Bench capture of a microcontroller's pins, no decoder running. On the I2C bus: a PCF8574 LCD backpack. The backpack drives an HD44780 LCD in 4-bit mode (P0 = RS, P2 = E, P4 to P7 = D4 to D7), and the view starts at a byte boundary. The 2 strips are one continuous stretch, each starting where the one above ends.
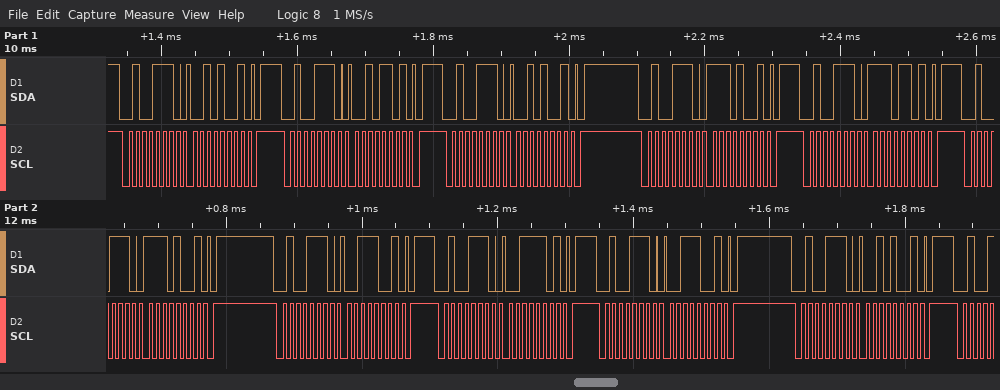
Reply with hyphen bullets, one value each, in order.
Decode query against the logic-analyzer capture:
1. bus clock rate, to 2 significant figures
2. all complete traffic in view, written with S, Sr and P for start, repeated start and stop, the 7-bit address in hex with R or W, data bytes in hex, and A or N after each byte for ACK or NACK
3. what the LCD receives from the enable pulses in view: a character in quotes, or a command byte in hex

- 100 kHz
- S 27W A 29 A P S 27W A 2D A P S 27W A 29 A P S 27W A E9 A P S 27W A ED A P S 27W A E9 A P S 27W A 39 A P S 27W A 3D A P S 27W A 39 A P S 27W A 29 A P
- '.'
